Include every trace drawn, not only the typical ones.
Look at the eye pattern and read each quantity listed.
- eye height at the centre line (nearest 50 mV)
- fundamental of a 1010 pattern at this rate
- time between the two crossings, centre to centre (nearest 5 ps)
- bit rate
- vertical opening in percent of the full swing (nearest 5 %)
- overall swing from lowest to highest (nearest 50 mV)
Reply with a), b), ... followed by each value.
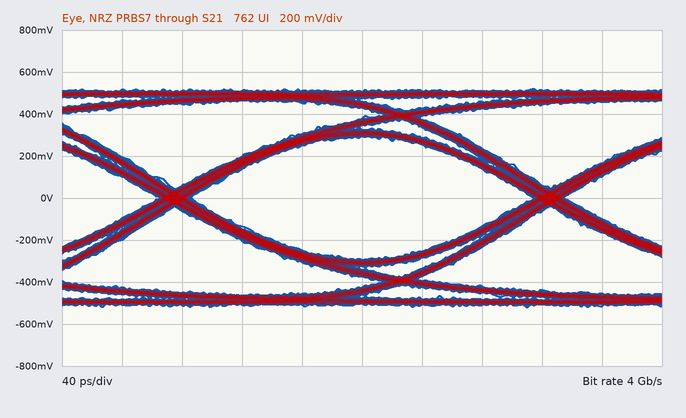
a) 600 mV
b) 2 GHz
c) 250 ps
d) 4 Gb/s
e) 55 %
f) 1.05 V
